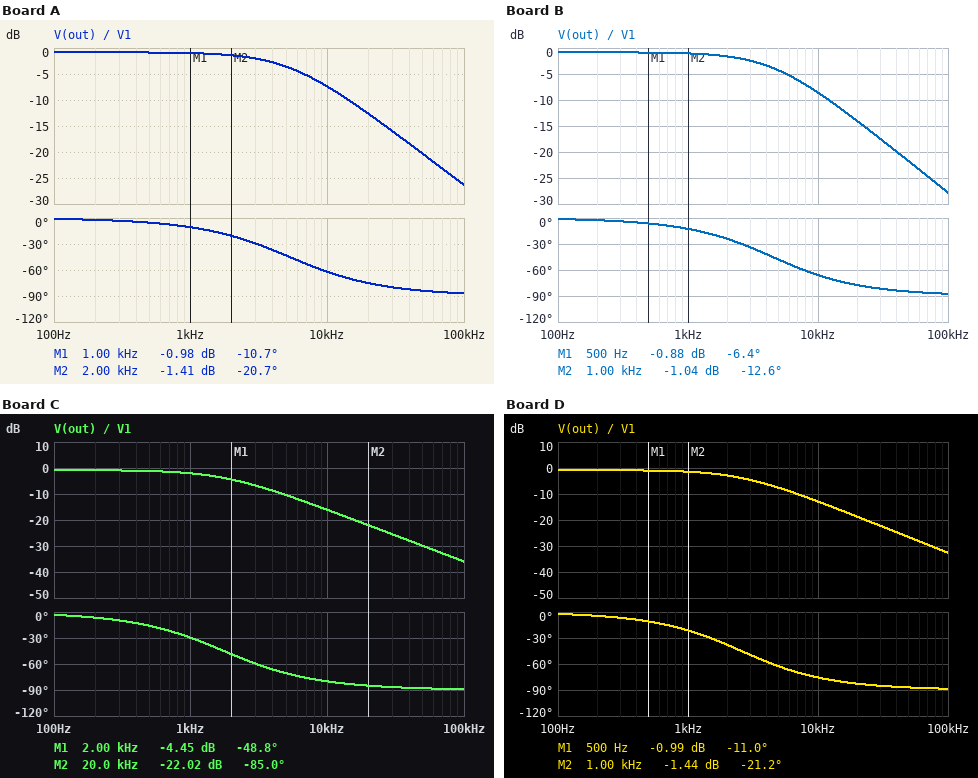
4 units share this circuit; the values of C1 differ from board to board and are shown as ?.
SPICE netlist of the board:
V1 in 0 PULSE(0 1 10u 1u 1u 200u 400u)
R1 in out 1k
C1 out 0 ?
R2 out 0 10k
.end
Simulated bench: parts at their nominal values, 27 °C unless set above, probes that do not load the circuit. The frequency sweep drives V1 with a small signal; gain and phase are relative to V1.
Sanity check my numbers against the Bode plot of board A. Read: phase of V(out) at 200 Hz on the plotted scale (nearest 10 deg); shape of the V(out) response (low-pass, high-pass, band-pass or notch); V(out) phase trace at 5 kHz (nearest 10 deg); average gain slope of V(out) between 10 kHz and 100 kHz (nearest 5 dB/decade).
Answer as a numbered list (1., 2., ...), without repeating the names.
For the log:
1. 0 deg
2. low-pass
3. -40 deg
4. -20 dB/decade
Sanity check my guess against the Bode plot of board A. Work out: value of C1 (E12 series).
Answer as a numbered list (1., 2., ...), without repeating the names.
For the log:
1. 33 nF
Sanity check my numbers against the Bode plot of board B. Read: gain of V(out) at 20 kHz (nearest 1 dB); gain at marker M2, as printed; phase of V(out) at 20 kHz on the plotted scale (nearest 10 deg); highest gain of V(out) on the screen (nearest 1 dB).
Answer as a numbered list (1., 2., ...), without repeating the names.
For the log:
1. -14 dB
2. -1.04 dB
3. -80 deg
4. -1 dB
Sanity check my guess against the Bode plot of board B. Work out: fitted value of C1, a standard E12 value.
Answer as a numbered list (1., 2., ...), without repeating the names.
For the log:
1. 39 nF
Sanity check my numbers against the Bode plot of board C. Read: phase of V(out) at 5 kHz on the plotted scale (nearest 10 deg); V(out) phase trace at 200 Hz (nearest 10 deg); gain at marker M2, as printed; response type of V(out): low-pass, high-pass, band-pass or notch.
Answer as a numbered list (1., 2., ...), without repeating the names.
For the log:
1. -70 deg
2. -10 deg
3. -22.02 dB
4. low-pass
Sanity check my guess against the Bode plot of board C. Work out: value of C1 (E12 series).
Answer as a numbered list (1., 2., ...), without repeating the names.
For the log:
1. 100 nF
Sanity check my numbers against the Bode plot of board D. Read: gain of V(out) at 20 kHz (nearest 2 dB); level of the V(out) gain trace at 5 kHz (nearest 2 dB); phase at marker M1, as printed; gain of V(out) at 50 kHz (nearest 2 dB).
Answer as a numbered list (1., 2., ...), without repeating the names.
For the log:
1. -18 dB
2. -8 dB
3. -11.0 deg
4. -26 dB
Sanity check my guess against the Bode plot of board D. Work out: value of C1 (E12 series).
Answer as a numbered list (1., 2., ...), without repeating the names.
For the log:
1. 68 nF
